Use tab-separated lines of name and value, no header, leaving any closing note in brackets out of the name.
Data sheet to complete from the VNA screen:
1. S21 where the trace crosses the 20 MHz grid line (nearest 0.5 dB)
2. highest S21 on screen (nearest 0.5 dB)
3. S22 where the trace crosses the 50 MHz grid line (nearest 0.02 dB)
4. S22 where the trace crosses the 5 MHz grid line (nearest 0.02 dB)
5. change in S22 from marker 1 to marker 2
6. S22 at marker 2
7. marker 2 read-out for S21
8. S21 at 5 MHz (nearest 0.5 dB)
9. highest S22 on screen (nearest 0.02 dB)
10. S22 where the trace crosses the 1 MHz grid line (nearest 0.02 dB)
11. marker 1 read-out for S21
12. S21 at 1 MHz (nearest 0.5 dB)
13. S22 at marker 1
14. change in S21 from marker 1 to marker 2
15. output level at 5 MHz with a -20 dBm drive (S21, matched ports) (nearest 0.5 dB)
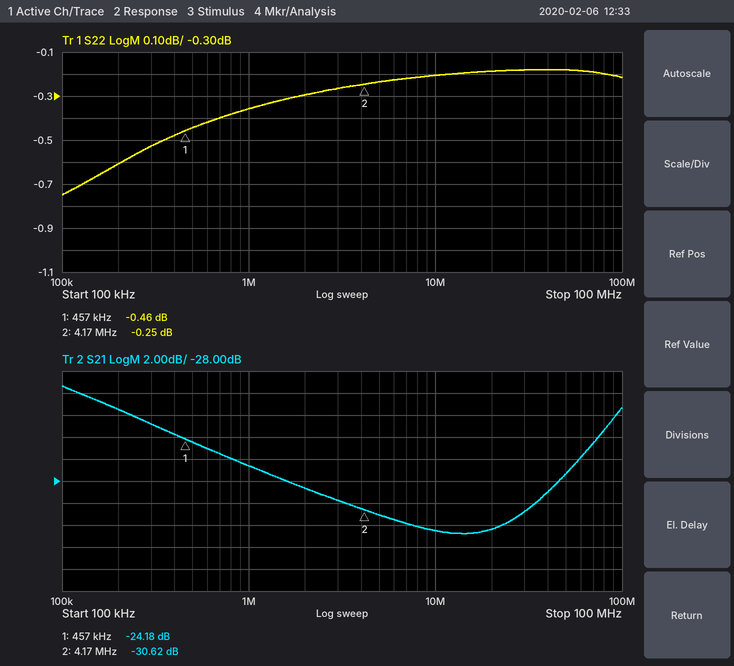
S21 where the trace crosses the 20 MHz grid line	-32.5 dB
highest S21 on screen	-19.5 dB
S22 where the trace crosses the 50 MHz grid line	-0.18 dB
S22 where the trace crosses the 5 MHz grid line	-0.24 dB
change in S22 from marker 1 to marker 2	0.21 dB
S22 at marker 2	-0.25 dB
marker 2 read-out for S21	-30.62 dB
S21 at 5 MHz	-31.0 dB
highest S22 on screen	-0.18 dB
S22 where the trace crosses the 1 MHz grid line	-0.36 dB
marker 1 read-out for S21	-24.18 dB
S21 at 1 MHz	-26.5 dB
S22 at marker 1	-0.46 dB
change in S21 from marker 1 to marker 2	-6.44 dB
output level at 5 MHz with a -20 dBm drive (S21, matched ports)	-51.0 dBm
